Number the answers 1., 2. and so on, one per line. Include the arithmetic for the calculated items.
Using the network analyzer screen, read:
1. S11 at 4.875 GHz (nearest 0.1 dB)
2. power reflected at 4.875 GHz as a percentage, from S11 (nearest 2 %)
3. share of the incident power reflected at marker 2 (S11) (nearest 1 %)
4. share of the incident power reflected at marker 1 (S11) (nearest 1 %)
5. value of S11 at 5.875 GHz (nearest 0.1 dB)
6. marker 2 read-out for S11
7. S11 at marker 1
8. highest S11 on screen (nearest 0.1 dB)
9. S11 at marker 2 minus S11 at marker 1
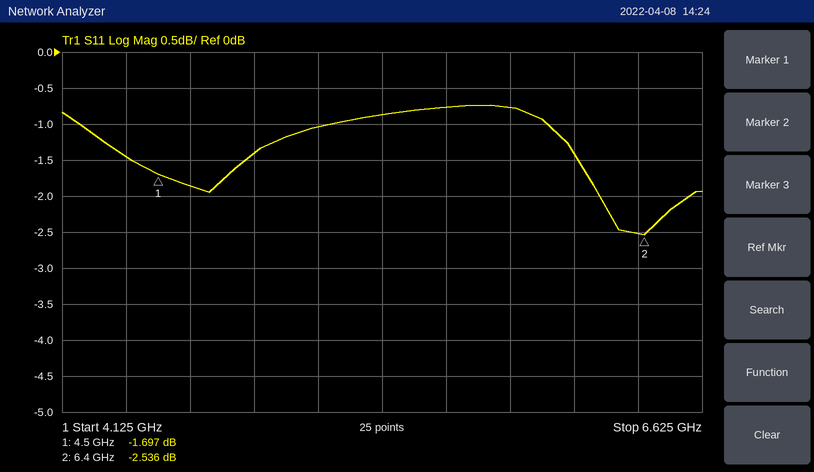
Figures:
1. -1.4 dB
2. 10^(-1.4/10) ≈ 72 %
3. 10^(-2.536/10) ≈ 56 %
4. 10^(-1.697/10) ≈ 68 %
5. -0.8 dB
6. -2.536 dB
7. -1.697 dB
8. -0.7 dB
9. -2.536 − (-1.697) = -0.839 dB
